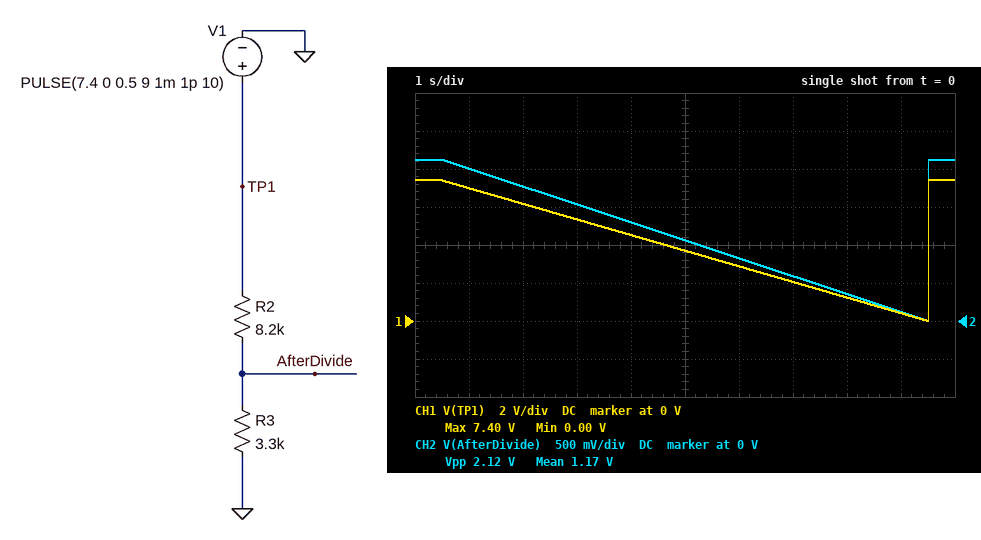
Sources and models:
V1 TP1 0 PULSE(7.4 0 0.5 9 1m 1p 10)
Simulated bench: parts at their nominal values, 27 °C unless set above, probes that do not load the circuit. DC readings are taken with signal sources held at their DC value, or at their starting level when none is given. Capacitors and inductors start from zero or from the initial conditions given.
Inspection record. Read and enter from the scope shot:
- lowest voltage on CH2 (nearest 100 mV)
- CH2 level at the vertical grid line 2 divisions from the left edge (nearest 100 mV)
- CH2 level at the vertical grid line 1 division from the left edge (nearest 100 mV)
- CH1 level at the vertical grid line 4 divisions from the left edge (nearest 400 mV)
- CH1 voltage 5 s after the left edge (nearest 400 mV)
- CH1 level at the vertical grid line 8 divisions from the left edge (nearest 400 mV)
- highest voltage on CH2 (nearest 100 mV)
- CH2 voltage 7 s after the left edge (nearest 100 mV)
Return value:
0 V
1.8 V
2.0 V
4.4 V
3.6 V
1.2 V
2.1 V
600 mV
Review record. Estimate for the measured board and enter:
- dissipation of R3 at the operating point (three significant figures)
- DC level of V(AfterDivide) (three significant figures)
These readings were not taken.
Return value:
1.37 mW
2.12 V
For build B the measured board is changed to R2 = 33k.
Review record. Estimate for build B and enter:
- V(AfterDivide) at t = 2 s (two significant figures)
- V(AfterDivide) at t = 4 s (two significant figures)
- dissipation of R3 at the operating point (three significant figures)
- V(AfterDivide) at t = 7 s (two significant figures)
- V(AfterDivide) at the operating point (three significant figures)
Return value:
560 mV
410 mV
137 µW
190 mV
673 mV
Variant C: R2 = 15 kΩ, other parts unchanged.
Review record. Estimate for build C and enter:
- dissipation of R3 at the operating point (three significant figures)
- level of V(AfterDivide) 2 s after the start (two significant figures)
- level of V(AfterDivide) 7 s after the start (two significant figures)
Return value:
540 µW
1.1 V
370 mV
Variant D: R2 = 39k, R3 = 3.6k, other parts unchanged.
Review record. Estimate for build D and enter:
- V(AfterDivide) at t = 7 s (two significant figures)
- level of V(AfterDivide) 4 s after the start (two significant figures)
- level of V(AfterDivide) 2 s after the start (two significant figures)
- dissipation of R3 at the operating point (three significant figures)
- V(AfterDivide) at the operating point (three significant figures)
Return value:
170 mV
380 mV
520 mV
109 µW
625 mV
